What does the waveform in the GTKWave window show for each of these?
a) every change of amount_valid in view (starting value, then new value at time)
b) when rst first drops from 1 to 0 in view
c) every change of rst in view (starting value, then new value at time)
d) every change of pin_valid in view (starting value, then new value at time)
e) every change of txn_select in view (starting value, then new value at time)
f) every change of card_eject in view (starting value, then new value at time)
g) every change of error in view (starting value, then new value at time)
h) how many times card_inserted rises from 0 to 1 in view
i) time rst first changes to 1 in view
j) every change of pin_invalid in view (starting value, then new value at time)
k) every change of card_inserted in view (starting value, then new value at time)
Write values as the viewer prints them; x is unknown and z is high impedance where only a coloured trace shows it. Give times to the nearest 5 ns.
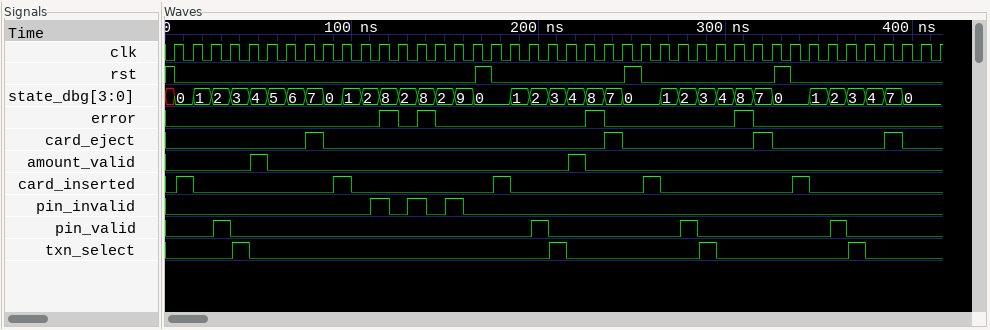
0, 1 at 45 ns, 0 at 55 ns, 1 at 215 ns, 0 at 225 ns
5 ns
1, 0 at 5 ns, 1 at 165 ns, 0 at 175 ns, 1 at 245 ns, 0 at 255 ns, 1 at 325 ns, 0 at 335 ns
0, 1 at 25 ns, 0 at 35 ns, 1 at 195 ns, 0 at 205 ns, 1 at 275 ns, 0 at 285 ns, 1 at 355 ns, 0 at 365 ns
0, 1 at 35 ns, 0 at 45 ns, 1 at 205 ns, 0 at 215 ns, 1 at 285 ns, 0 at 295 ns, 1 at 365 ns, 0 at 375 ns
0, 1 at 75 ns, 0 at 85 ns, 1 at 235 ns, 0 at 245 ns, 1 at 315 ns, 0 at 325 ns, 1 at 385 ns, 0 at 395 ns
0, 1 at 115 ns, 0 at 125 ns, 1 at 135 ns, 0 at 145 ns, 1 at 225 ns, 0 at 235 ns, 1 at 305 ns, 0 at 315 ns
5
165 ns
0, 1 at 110 ns, 0 at 120 ns, 1 at 130 ns, 0 at 140 ns, 1 at 150 ns, 0 at 160 ns
0, 1 at 5 ns, 0 at 15 ns, 1 at 90 ns, 0 at 100 ns, 1 at 175 ns, 0 at 185 ns, 1 at 255 ns, 0 at 265 ns, 1 at 335 ns, 0 at 345 ns
